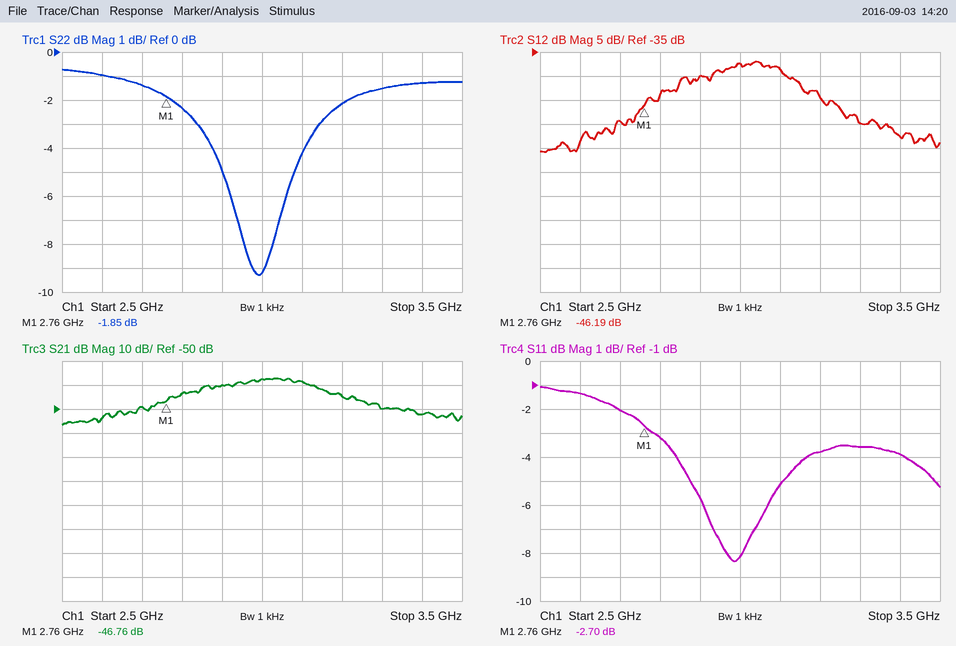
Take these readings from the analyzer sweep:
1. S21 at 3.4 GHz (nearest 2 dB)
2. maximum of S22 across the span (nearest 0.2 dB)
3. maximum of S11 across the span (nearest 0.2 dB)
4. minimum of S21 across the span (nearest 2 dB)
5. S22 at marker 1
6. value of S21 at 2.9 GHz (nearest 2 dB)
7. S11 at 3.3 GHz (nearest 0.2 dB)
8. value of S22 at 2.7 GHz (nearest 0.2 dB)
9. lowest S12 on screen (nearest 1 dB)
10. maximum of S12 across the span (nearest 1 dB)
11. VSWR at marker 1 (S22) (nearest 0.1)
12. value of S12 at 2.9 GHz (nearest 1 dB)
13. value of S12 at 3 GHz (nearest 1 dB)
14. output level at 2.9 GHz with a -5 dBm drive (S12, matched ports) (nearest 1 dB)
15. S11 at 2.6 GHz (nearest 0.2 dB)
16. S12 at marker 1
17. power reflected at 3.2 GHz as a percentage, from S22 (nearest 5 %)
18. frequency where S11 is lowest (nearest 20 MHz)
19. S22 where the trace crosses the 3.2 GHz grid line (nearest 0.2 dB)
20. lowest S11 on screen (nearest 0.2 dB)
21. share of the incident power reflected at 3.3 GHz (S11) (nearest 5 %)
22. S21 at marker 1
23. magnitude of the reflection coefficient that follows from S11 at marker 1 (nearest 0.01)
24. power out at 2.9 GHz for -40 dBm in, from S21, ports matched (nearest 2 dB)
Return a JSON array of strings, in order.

["-52 dB", "-0.8 dB", "-1.0 dB", "-56 dB", "-1.85 dB", "-40 dB", "-3.6 dB", "-1.4 dB", "-56 dB", "-37 dB", "9.4", "-40 dB", "-37 dB", "-45 dBm", "-1.4 dB", "-46.19 dB", "60 %", "2.98 GHz", "-2.2 dB", "-8.4 dB", "45 %", "-46.76 dB", "0.73", "-80 dBm"]
